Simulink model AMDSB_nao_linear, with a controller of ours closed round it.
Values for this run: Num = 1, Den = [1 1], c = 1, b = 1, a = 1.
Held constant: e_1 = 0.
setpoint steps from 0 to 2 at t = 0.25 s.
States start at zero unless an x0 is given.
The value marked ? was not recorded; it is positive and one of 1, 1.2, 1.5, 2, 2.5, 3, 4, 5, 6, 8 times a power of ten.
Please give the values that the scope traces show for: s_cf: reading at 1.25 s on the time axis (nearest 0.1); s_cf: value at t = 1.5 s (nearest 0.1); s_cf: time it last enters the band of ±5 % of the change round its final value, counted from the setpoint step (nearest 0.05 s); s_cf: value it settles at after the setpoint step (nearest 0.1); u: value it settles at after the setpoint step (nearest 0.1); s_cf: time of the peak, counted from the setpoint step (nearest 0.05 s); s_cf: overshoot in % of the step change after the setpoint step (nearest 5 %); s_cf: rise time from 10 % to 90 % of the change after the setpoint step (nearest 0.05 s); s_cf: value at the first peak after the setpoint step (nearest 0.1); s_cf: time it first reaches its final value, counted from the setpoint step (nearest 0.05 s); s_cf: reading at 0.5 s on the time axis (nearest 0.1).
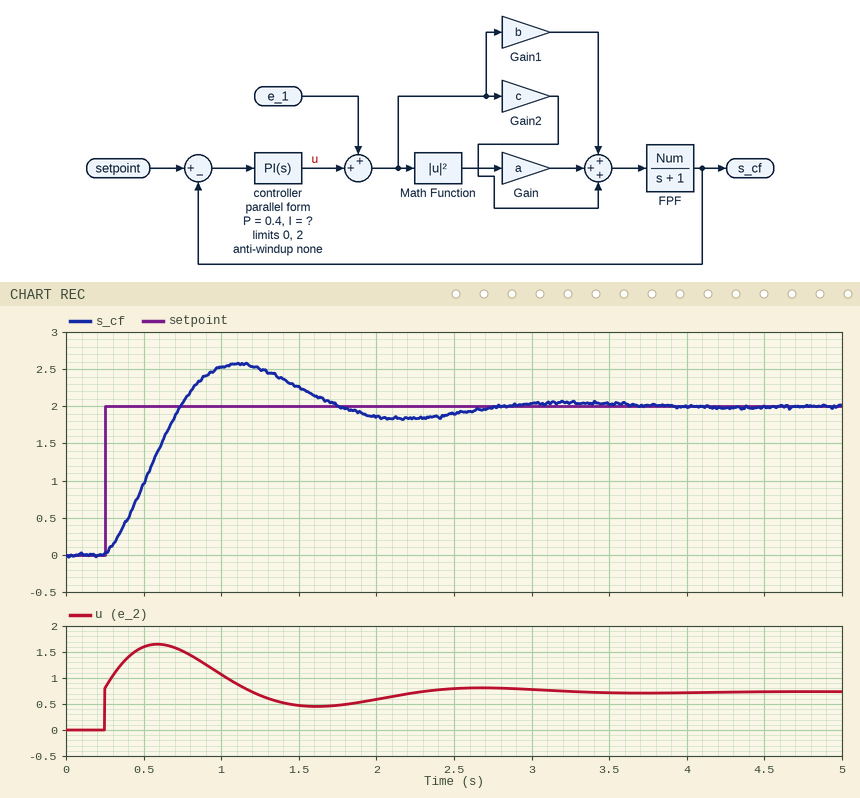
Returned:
2.5
2.3
2.25 s
2.0
0.7
0.85 s
30 %
0.35 s
2.6
0.50 s
1.0
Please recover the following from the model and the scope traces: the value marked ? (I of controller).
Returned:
3
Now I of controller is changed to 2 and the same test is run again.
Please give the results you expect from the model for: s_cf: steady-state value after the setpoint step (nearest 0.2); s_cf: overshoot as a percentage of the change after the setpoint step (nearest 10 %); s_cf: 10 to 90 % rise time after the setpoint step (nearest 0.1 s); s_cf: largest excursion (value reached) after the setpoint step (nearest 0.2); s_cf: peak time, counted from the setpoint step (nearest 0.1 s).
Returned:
2.0
20 %
0.5 s
2.4
1.1 s
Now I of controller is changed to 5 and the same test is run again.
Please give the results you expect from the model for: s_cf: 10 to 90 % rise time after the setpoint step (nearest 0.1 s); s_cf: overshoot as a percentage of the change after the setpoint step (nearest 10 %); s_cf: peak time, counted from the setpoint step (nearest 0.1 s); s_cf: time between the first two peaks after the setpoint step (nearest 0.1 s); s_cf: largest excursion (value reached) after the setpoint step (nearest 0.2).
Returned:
0.3 s
40 %
0.6 s
1.6 s
2.8
